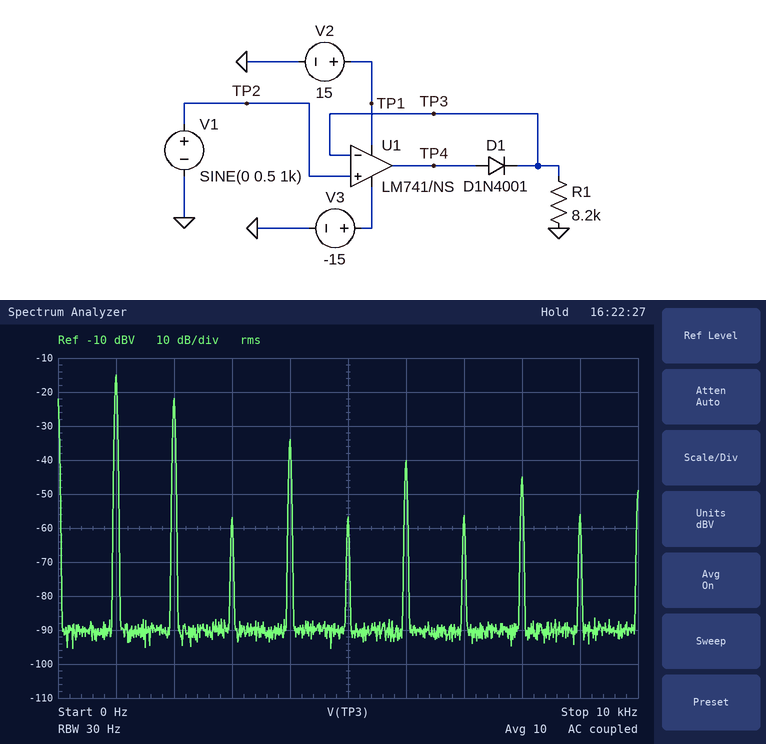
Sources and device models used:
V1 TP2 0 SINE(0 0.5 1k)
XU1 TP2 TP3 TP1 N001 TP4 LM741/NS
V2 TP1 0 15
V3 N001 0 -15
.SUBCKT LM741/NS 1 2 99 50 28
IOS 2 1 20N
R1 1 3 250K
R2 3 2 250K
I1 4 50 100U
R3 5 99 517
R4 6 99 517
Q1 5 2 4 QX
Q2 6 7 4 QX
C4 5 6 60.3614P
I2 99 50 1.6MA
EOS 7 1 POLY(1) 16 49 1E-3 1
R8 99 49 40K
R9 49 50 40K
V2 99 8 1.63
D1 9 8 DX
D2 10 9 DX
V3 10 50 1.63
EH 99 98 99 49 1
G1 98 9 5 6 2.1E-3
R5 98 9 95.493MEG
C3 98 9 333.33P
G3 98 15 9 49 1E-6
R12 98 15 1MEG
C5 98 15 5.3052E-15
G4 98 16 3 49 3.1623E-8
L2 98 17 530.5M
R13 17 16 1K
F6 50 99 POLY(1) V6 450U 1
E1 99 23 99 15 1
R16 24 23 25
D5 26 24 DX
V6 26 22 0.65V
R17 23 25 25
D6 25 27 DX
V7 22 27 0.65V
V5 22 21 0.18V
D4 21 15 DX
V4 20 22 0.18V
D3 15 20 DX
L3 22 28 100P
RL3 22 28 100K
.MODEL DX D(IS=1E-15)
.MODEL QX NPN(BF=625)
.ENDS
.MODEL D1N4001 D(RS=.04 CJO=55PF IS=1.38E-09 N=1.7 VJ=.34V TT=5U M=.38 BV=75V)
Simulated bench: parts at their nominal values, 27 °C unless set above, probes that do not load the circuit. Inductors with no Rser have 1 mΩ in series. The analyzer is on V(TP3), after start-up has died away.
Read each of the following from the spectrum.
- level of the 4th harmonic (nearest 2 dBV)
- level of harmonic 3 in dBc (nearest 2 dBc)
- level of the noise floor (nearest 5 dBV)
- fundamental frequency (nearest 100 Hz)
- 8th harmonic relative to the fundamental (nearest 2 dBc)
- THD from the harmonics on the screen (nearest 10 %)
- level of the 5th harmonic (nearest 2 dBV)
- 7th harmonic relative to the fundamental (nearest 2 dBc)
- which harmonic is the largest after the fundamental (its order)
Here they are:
-34 dBV
-42 dBc
-90 dBV
1.0 kHz
-30 dBc
50 %
-56 dBV
-42 dBc
2
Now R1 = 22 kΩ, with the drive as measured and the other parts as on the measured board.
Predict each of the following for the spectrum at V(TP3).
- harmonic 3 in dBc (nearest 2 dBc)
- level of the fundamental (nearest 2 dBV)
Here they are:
-32 dBc
-14 dBV
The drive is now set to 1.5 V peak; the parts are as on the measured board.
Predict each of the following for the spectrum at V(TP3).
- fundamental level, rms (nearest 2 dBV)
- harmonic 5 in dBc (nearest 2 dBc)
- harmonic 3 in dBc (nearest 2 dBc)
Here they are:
-6 dBV
-36 dBc
-36 dBc
